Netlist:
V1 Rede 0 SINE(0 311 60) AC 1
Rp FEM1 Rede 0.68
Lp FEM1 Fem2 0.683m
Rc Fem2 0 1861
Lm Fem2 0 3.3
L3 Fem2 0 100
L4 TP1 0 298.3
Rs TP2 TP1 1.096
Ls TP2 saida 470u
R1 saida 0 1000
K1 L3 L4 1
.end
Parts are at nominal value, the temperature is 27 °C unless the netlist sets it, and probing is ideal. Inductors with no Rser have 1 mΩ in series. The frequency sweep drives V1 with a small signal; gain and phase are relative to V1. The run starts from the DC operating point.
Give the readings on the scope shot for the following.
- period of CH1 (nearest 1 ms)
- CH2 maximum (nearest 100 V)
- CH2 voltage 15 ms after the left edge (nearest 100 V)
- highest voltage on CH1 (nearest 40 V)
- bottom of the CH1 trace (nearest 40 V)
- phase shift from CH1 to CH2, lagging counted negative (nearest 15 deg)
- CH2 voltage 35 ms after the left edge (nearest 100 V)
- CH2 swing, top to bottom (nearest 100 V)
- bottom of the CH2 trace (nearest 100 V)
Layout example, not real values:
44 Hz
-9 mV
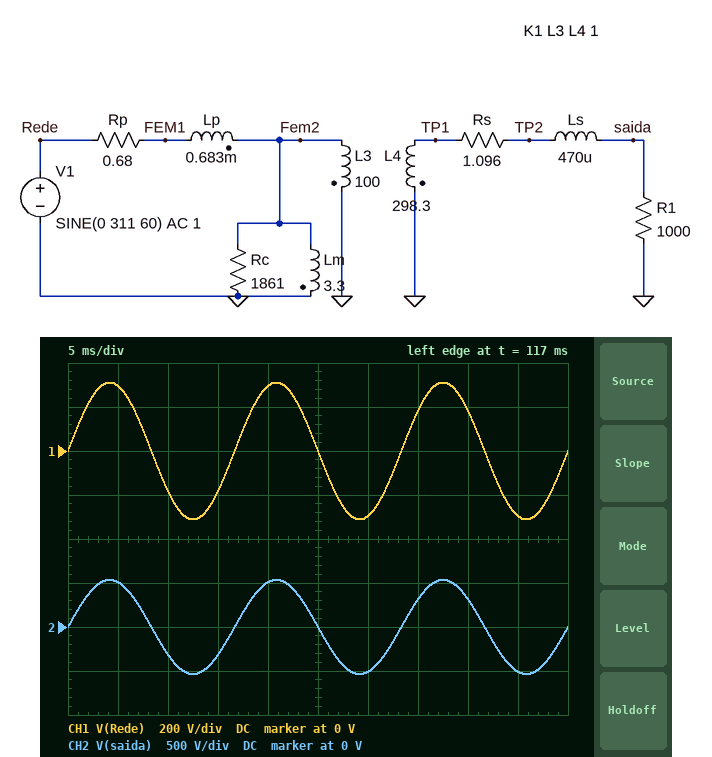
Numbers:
17 ms
500 V
-300 V
320 V
-320 V
0 deg
300 V
1.1 kV
-500 V
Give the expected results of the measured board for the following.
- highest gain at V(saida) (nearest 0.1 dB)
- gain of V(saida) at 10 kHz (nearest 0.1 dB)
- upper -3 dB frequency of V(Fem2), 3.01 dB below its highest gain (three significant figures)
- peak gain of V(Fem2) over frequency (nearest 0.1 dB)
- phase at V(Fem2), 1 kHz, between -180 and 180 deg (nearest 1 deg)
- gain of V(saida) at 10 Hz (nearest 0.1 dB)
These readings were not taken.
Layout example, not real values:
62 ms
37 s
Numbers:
4.7 dB
4.6 dB
58.4 kHz
0 dB
-1 deg
4.7 dB
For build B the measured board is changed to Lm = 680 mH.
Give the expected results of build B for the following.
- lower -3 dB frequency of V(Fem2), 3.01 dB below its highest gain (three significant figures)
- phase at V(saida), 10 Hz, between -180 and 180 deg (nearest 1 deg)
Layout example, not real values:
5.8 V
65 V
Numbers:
160 mHz
1 deg
